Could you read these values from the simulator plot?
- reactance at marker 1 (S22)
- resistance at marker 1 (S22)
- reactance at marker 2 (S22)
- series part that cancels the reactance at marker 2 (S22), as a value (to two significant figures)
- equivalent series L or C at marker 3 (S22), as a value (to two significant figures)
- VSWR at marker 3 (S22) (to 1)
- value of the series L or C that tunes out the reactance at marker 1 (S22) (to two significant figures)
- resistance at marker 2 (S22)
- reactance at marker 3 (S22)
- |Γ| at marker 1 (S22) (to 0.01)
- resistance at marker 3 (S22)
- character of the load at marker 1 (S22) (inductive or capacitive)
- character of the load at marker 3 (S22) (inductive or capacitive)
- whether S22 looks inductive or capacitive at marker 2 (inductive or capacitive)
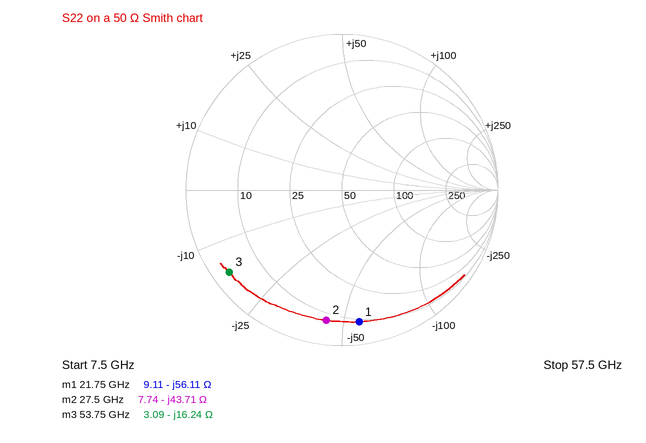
-56.11 Ω
9.11 Ω
-43.71 Ω
250 pH
180 fF
18
410 pH
7.74 Ω
-16.24 Ω
0.85
3.09 Ω
capacitive
capacitive
capacitive
